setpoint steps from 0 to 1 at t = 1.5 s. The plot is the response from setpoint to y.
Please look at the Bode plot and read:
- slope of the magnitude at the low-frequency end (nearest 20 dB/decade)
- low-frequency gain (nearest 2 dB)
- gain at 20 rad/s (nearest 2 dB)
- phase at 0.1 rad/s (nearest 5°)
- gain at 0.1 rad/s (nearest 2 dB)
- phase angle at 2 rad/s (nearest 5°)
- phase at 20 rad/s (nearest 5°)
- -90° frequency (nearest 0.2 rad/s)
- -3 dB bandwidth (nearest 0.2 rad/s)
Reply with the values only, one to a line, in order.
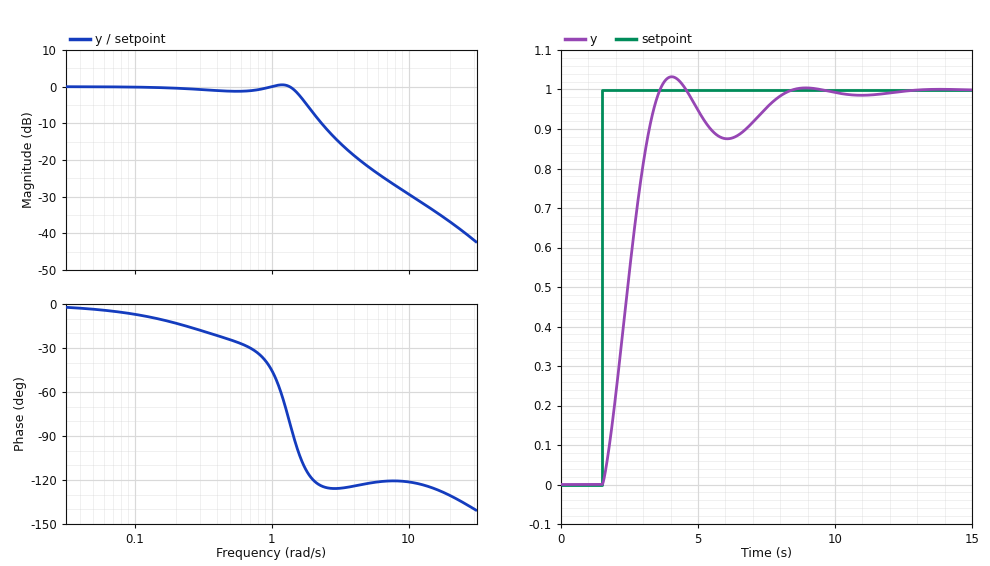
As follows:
0 dB/decade
0 dB
-36 dB
-5°
0 dB
-120°
-130°
1.4 rad/s
1.6 rad/s
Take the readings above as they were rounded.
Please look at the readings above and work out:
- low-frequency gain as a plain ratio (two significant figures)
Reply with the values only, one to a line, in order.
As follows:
1.0
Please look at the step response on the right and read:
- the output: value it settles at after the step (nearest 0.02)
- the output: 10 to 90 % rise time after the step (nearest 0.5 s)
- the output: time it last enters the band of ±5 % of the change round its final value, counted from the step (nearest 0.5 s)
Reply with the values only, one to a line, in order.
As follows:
1.00
1.5 s
6.0 s
